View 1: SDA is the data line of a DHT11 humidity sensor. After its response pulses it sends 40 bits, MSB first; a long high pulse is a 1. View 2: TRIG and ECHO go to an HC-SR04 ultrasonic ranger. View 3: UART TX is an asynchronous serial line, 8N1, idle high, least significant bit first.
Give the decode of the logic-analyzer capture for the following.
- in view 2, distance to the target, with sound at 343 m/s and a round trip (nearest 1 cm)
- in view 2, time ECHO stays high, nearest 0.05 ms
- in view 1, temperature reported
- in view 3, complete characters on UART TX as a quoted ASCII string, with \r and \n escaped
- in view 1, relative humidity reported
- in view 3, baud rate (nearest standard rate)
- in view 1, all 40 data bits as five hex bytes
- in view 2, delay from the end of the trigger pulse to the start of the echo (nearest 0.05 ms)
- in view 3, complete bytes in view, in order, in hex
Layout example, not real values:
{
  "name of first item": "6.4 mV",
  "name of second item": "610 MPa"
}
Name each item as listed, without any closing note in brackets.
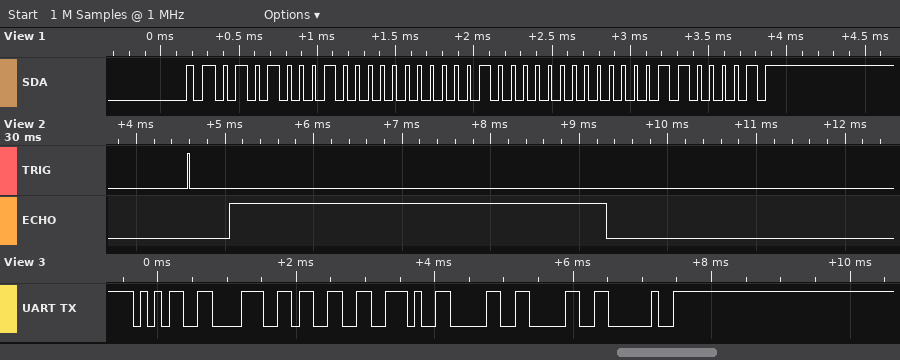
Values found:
{
  "in view 2, distance to the target, with sound at 343 m/s and a round trip": "73 cm",
  "in view 2, time ECHO stays high, nearest 0.05 ms": "4.25 ms",
  "in view 1, temperature reported": "16.0 °C",
  "in view 3, complete characters on UART TX as a quoted ASCII string, with \\r and \\n escaped": "\"583.00 \"",
  "in view 1, relative humidity reported": "81 %",
  "in view 3, baud rate": "9600 baud",
  "in view 1, all 40 data bits as five hex bytes": "51 00 10 00 61",
  "in view 2, delay from the end of the trigger pulse to the start of the echo": "0.45 ms",
  "in view 3, complete bytes in view, in order, in hex": "35 38 33 2E 30 30 20"
}
